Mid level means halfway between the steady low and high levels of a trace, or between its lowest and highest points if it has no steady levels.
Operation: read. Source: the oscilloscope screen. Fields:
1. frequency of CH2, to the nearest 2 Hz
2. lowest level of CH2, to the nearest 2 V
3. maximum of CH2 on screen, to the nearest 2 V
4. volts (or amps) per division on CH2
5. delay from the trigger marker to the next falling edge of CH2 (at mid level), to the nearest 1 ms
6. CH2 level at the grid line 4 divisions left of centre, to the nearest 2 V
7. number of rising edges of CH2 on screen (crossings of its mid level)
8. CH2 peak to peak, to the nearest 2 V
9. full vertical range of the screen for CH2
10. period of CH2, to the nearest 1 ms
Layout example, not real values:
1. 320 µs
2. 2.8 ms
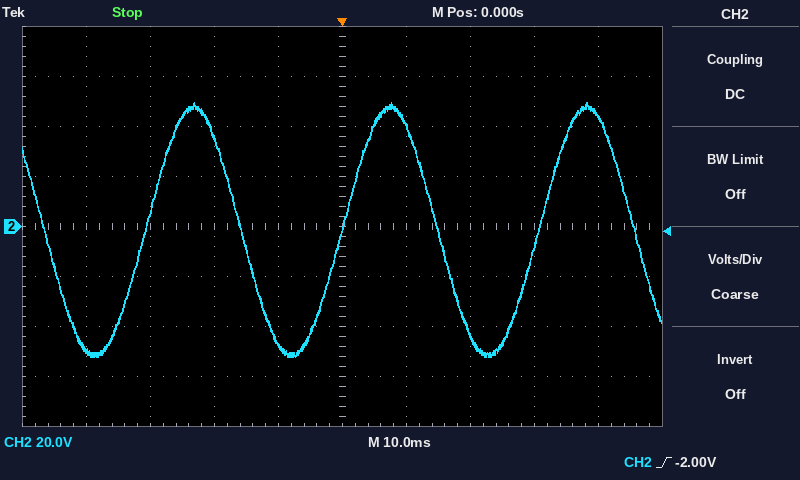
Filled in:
1. 32 Hz
2. -52 V
3. 50 V
4. 20 V
5. 15 ms
6. -50 V
7. 3
8. 102 V
9. 160 V
10. 31 ms
